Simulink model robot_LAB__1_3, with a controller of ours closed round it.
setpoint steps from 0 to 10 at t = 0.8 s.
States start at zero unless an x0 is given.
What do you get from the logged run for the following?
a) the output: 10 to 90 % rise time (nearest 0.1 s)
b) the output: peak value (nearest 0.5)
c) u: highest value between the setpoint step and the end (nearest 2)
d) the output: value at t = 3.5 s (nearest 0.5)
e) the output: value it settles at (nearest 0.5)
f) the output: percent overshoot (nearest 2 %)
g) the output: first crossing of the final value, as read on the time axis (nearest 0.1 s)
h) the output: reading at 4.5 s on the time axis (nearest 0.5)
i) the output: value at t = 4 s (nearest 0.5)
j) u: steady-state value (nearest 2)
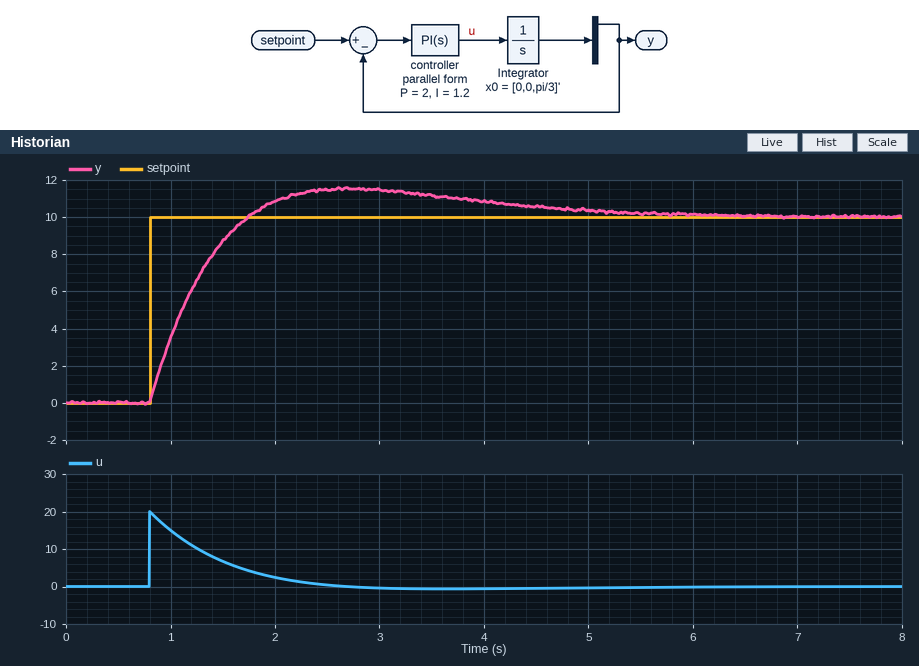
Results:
0.7 s
11.5
20
11.0
10.0
16 %
1.7 s
10.5
11.0
0
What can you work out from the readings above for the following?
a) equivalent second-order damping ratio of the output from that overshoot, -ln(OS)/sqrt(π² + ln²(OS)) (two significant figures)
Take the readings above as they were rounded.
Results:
0.50
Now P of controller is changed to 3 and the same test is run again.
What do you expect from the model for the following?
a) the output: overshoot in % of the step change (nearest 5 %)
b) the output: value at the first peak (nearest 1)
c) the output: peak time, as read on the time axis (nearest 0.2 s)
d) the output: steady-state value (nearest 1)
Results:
10 %
11
2.4 s
10
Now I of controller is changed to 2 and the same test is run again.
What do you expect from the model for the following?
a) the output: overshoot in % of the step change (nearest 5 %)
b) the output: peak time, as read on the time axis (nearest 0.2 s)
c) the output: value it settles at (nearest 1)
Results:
20 %
2.4 s
10
